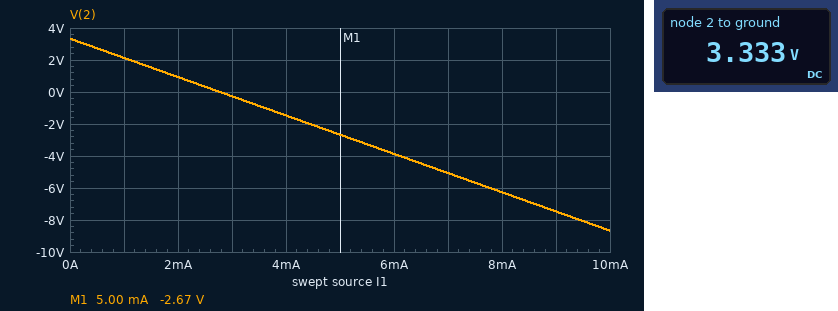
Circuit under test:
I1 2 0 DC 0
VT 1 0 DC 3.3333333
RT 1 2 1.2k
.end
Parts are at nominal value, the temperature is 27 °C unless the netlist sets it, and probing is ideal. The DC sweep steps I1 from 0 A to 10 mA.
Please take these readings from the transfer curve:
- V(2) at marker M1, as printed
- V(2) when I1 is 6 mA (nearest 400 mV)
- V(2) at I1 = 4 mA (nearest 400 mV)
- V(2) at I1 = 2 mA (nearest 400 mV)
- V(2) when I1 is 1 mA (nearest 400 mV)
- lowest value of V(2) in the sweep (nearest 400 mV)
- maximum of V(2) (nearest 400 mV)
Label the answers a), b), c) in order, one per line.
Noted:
a) -2.67 V
b) -4.0 V
c) -1.6 V
d) 800 mV
e) 2.0 V
f) -8.8 V
g) 3.2 V
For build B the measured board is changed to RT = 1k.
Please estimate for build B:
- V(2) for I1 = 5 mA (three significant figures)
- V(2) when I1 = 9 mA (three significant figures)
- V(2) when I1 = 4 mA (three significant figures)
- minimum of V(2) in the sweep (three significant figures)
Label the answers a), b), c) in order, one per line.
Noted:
a) -1.67 V
b) -5.67 V
c) -667 mV
d) -6.67 V
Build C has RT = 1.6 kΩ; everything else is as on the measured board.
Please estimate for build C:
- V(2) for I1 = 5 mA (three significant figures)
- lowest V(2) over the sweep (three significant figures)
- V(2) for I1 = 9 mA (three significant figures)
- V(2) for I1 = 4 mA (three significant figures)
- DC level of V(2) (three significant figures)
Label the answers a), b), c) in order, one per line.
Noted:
a) -4.67 V
b) -12.7 V
c) -11.1 V
d) -3.07 V
e) 3.33 V
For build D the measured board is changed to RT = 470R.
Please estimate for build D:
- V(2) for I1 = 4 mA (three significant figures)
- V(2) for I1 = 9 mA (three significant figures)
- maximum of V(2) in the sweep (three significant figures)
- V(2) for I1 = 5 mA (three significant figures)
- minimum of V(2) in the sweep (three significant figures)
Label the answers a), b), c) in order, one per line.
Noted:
a) 1.45 V
b) -897 mV
c) 3.33 V
d) 983 mV
e) -1.37 V
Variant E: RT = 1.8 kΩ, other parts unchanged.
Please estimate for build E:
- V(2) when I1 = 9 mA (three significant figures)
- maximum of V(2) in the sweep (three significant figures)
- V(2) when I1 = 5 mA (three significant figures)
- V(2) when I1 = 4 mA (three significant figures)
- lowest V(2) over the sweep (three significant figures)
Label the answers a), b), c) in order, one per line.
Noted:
a) -12.9 V
b) 3.33 V
c) -5.67 V
d) -3.87 V
e) -14.7 V
